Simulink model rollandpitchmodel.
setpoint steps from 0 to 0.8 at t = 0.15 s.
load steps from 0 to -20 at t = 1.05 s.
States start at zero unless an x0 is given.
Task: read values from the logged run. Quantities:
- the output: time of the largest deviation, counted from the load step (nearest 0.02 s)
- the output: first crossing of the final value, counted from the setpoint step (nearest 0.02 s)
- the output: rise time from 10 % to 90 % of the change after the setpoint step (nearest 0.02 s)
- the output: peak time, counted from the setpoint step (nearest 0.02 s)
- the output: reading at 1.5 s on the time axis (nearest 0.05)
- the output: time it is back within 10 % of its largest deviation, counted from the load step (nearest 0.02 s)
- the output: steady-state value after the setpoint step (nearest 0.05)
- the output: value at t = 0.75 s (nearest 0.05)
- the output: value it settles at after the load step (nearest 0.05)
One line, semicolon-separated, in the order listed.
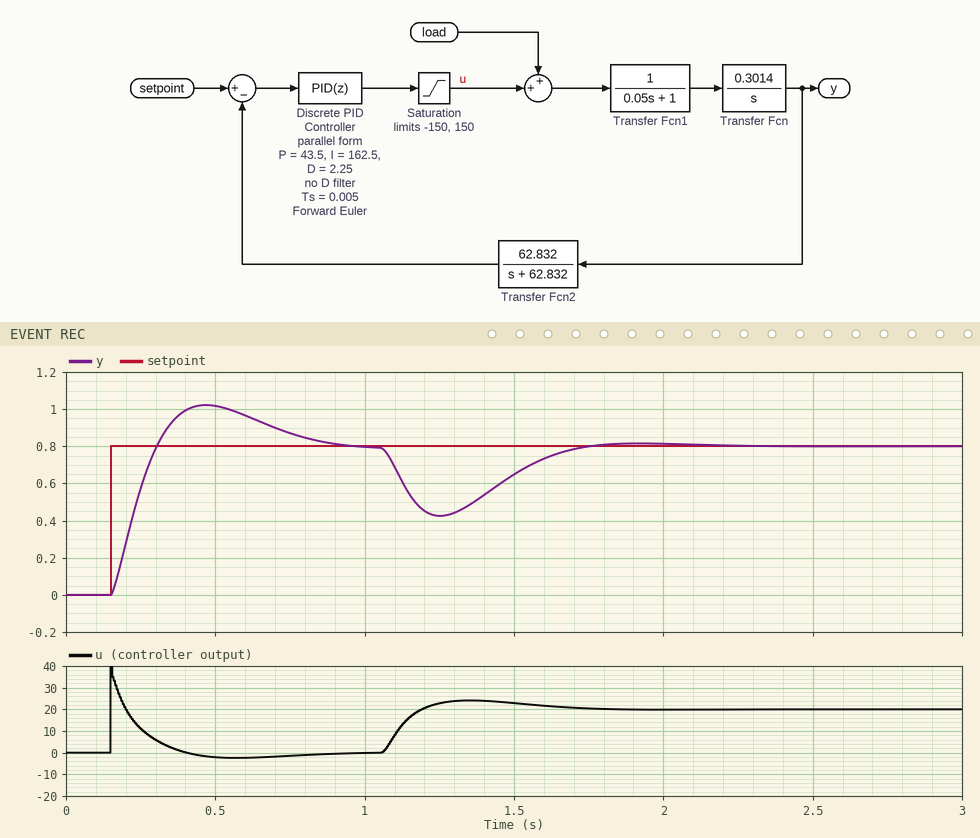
0.20 s; 0.16 s; 0.12 s; 0.32 s; 0.65; 0.60 s; 0.80; 0.85; 0.80
